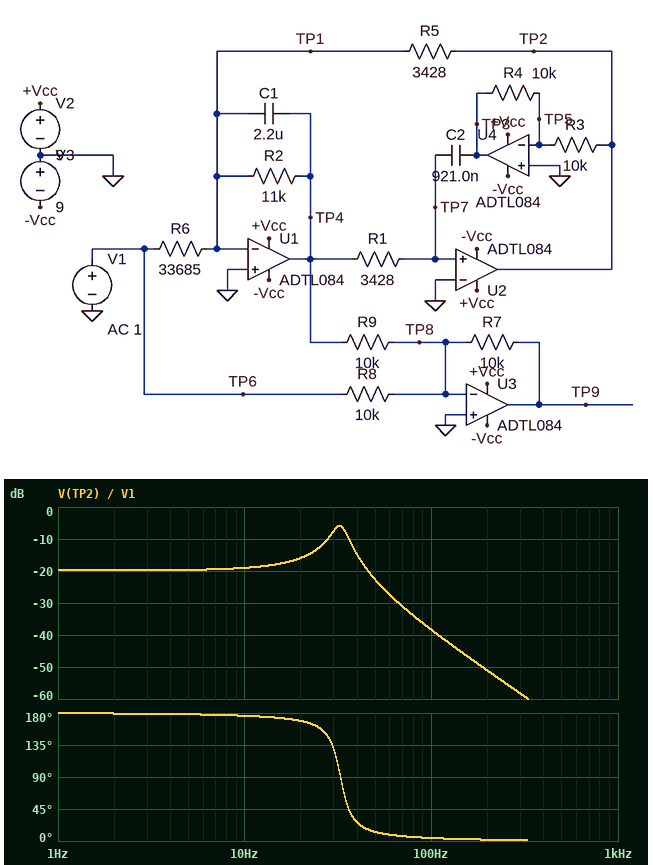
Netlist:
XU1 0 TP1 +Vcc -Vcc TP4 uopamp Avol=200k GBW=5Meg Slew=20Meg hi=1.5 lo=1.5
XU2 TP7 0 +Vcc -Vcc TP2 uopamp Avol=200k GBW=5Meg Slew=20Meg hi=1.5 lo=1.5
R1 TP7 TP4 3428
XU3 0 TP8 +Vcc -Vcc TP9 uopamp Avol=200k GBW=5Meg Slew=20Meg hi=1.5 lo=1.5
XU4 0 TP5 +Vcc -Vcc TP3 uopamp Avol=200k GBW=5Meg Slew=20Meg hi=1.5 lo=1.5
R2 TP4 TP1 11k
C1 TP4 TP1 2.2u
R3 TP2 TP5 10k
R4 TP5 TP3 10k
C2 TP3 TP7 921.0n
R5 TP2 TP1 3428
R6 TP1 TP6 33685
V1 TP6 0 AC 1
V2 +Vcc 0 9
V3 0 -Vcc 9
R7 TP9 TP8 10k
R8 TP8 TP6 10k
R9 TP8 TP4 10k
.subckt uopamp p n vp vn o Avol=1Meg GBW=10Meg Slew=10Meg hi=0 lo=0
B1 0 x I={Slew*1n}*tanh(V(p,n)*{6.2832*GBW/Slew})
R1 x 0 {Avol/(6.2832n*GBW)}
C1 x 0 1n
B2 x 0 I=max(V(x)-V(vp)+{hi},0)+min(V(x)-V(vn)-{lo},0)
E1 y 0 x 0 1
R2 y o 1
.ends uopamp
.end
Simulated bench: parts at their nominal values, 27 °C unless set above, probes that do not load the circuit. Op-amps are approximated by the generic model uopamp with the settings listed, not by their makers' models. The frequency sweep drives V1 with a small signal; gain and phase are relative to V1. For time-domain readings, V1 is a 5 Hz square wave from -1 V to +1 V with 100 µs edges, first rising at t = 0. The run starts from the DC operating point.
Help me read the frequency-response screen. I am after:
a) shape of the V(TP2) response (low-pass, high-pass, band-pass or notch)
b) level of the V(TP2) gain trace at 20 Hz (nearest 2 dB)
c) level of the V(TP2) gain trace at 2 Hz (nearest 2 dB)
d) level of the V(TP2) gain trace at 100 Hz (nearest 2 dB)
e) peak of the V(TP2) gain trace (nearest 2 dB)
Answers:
low-pass
-16 dB
-20 dB
-38 dB
-6 dB
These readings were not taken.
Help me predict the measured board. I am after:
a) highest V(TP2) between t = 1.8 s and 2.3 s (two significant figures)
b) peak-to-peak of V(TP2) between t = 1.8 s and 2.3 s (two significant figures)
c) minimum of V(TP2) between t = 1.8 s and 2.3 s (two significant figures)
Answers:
250 mV
490 mV
-250 mV
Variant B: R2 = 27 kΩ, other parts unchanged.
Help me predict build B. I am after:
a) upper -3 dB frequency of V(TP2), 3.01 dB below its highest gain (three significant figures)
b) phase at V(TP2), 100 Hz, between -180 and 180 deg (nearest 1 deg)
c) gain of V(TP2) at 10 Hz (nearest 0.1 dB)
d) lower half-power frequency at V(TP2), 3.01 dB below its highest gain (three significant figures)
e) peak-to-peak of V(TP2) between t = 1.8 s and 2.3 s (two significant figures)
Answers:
33.9 Hz
2 deg
-19.0 dB
31.2 Hz
530 mV
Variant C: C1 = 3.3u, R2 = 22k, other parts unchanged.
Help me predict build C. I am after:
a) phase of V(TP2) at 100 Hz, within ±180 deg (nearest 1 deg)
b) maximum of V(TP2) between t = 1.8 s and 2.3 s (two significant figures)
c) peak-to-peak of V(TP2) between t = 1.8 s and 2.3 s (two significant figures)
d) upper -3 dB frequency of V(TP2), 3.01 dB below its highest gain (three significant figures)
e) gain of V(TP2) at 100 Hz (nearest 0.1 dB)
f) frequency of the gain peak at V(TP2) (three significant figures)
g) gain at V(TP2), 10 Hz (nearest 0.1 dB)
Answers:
1 deg
320 mV
640 mV
27.7 Hz
-42.2 dB
26.6 Hz
-18.5 dB
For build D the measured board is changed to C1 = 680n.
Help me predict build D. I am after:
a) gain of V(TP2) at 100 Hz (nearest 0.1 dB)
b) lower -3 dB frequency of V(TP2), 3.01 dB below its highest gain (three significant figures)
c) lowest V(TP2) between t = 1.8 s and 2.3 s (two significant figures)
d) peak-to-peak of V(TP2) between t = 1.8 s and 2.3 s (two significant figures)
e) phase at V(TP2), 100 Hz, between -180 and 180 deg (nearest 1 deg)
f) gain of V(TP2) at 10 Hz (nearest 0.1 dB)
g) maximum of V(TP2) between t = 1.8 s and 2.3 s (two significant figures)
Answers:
-25.9 dB
44.6 Hz
-220 mV
430 mV
18 deg
-19.6 dB
220 mV
